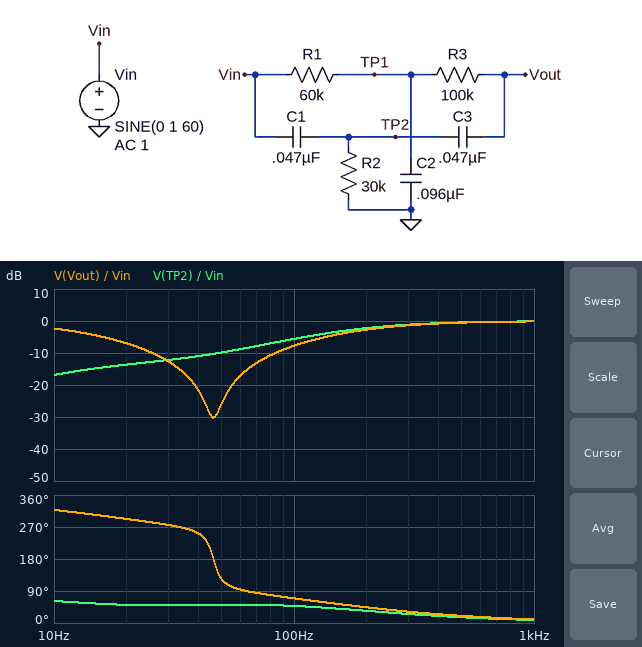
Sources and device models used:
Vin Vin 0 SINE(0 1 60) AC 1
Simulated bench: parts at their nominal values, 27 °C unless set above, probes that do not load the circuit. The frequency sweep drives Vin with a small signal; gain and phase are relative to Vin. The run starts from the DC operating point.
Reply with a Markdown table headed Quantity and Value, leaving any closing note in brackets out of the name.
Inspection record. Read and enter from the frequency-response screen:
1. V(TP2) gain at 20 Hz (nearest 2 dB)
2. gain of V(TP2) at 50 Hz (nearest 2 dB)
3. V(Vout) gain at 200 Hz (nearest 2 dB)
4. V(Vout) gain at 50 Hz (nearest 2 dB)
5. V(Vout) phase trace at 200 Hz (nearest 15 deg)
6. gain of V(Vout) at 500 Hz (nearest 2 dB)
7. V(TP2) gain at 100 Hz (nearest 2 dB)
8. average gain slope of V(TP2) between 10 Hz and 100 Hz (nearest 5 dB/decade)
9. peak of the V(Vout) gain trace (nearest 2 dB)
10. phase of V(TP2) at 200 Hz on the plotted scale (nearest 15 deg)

| Quantity | Value |
|---|---|
| V(TP2) gain at 20 Hz | -14 dB |
| gain of V(TP2) at 50 Hz | -10 dB |
| V(Vout) gain at 200 Hz | -2 dB |
| V(Vout) gain at 50 Hz | -26 dB |
| V(Vout) phase trace at 200 Hz | 45 deg |
| gain of V(Vout) at 500 Hz | 0 dB |
| V(TP2) gain at 100 Hz | -6 dB |
| average gain slope of V(TP2) between 10 Hz and 100 Hz | 10 dB/decade |
| peak of the V(Vout) gain trace | 0 dB |
| phase of V(TP2) at 200 Hz on the plotted scale | 30 deg |
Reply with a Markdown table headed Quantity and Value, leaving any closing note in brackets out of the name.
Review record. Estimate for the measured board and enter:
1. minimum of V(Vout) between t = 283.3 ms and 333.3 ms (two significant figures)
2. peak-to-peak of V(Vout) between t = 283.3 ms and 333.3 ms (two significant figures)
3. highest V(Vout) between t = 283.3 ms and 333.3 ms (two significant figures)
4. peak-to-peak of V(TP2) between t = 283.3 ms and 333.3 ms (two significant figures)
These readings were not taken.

| Quantity | Value |
|---|---|
| minimum of V(Vout) between t = 283.3 ms and 333.3 ms | -140 mV |
| peak-to-peak of V(Vout) between t = 283.3 ms and 333.3 ms | 280 mV |
| highest V(Vout) between t = 283.3 ms and 333.3 ms | 140 mV |
| peak-to-peak of V(TP2) between t = 283.3 ms and 333.3 ms | 730 mV |
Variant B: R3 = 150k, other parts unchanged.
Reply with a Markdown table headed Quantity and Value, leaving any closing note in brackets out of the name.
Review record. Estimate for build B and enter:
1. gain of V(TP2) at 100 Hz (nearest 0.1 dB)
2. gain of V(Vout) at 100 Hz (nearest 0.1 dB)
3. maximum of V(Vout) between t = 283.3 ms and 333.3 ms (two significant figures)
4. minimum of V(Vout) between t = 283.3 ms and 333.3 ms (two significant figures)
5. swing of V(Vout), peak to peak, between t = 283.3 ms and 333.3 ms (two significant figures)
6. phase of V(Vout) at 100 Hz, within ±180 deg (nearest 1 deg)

| Quantity | Value |
|---|---|
| gain of V(TP2) at 100 Hz | -5.0 dB |
| gain of V(Vout) at 100 Hz | -6.2 dB |
| maximum of V(Vout) between t = 283.3 ms and 333.3 ms | 230 mV |
| minimum of V(Vout) between t = 283.3 ms and 333.3 ms | -230 mV |
| swing of V(Vout), peak to peak, between t = 283.3 ms and 333.3 ms | 450 mV |
| phase of V(Vout) at 100 Hz, within ±180 deg | 65 deg |
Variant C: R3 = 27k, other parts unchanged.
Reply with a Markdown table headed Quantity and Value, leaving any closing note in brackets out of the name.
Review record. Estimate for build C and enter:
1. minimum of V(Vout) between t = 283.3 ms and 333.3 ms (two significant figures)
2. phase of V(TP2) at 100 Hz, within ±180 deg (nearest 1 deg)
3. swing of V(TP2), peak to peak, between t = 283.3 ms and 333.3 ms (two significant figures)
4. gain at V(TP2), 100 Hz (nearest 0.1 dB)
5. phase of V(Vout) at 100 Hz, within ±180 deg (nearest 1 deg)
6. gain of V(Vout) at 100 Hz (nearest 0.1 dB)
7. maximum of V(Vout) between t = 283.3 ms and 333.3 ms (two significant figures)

| Quantity | Value |
|---|---|
| minimum of V(Vout) between t = 283.3 ms and 333.3 ms | -100 mV |
| phase of V(TP2) at 100 Hz, within ±180 deg | 35 deg |
| swing of V(TP2), peak to peak, between t = 283.3 ms and 333.3 ms | 770 mV |
| gain at V(TP2), 100 Hz | -6.6 dB |
| phase of V(Vout) at 100 Hz, within ±180 deg | 59 deg |
| gain of V(Vout) at 100 Hz | -18.0 dB |
| maximum of V(Vout) between t = 283.3 ms and 333.3 ms | 100 mV |
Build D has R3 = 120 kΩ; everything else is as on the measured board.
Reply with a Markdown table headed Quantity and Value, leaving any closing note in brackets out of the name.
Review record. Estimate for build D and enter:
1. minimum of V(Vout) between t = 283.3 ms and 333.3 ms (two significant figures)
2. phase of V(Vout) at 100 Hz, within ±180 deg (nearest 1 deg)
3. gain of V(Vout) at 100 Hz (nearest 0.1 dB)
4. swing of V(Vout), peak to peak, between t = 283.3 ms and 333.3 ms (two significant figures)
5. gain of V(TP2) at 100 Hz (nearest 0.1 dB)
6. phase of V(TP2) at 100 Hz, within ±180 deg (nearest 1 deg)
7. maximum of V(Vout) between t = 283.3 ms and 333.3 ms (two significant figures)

| Quantity | Value |
|---|---|
| minimum of V(Vout) between t = 283.3 ms and 333.3 ms | -180 mV |
| phase of V(Vout) at 100 Hz, within ±180 deg | 67 deg |
| gain of V(Vout) at 100 Hz | -7.0 dB |
| swing of V(Vout), peak to peak, between t = 283.3 ms and 333.3 ms | 360 mV |
| gain of V(TP2) at 100 Hz | -5.3 dB |
| phase of V(TP2) at 100 Hz, within ±180 deg | 49 deg |
| maximum of V(Vout) between t = 283.3 ms and 333.3 ms | 180 mV |
